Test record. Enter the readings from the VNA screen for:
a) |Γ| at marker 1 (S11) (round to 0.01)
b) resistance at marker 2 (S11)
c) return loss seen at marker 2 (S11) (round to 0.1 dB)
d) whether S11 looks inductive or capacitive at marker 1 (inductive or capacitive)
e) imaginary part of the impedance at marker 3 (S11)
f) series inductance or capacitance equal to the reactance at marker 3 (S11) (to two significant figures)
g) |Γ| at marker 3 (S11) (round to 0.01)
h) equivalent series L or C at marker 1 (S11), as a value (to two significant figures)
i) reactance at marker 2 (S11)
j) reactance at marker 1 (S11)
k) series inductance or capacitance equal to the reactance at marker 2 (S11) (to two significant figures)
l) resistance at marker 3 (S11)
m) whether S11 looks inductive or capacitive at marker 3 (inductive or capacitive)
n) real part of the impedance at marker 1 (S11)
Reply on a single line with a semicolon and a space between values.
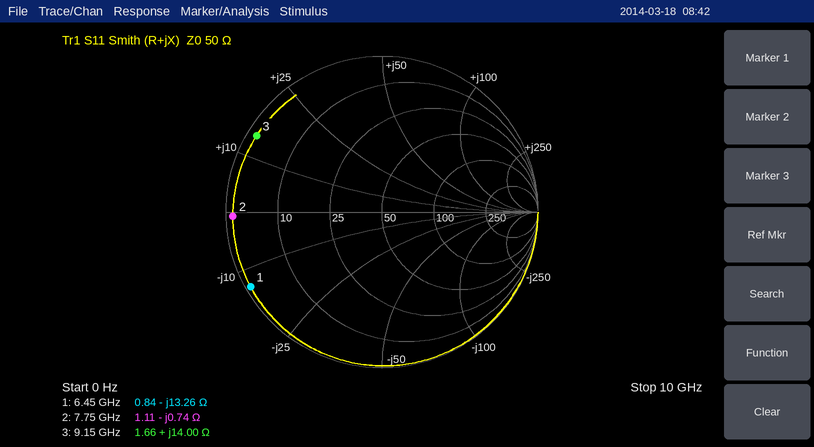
0.97; 1.11 Ω; 0.4 dB; capacitive; +14.00 Ω; 240 pH; 0.94; 1.9 pF; -0.74 Ω; -13.26 Ω; 28 pF; 1.66 Ω; inductive; 0.84 Ω
